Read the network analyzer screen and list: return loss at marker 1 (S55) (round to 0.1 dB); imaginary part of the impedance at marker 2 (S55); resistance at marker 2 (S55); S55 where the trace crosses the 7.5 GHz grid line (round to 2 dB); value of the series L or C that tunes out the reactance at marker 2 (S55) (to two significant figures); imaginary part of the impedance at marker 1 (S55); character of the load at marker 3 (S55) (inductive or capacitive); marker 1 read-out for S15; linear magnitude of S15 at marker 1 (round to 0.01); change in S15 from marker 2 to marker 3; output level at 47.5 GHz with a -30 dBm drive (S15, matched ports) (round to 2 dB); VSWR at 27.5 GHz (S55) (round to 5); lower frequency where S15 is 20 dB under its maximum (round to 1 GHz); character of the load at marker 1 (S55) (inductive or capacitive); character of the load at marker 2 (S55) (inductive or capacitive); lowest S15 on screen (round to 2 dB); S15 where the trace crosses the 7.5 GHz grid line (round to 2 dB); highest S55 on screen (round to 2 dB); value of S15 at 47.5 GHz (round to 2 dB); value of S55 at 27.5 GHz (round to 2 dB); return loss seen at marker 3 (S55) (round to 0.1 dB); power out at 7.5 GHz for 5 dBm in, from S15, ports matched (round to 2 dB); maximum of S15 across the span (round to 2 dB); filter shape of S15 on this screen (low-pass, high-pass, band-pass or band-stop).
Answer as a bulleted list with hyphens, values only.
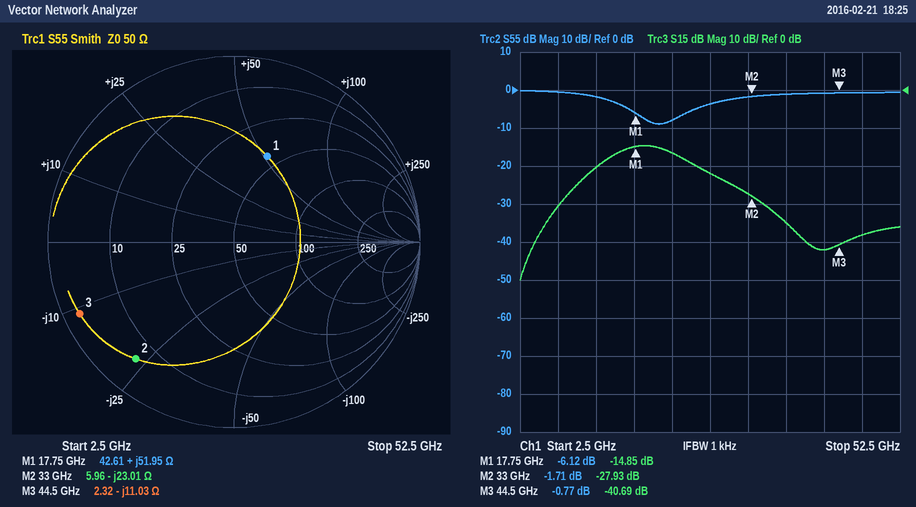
- 6.1 dB
- -23.01 Ω
- 5.96 Ω
- 0 dB
- 110 pH
- +51.95 Ω
- capacitive
- -14.85 dB
- 0.18
- -12.76 dB
- -68 dBm
- 5
- 6 GHz
- inductive
- capacitive
- -50 dB
- -30 dB
- 0 dB
- -38 dB
- -4 dB
- 0.8 dB
- -26 dBm
- -14 dB
- band-pass
